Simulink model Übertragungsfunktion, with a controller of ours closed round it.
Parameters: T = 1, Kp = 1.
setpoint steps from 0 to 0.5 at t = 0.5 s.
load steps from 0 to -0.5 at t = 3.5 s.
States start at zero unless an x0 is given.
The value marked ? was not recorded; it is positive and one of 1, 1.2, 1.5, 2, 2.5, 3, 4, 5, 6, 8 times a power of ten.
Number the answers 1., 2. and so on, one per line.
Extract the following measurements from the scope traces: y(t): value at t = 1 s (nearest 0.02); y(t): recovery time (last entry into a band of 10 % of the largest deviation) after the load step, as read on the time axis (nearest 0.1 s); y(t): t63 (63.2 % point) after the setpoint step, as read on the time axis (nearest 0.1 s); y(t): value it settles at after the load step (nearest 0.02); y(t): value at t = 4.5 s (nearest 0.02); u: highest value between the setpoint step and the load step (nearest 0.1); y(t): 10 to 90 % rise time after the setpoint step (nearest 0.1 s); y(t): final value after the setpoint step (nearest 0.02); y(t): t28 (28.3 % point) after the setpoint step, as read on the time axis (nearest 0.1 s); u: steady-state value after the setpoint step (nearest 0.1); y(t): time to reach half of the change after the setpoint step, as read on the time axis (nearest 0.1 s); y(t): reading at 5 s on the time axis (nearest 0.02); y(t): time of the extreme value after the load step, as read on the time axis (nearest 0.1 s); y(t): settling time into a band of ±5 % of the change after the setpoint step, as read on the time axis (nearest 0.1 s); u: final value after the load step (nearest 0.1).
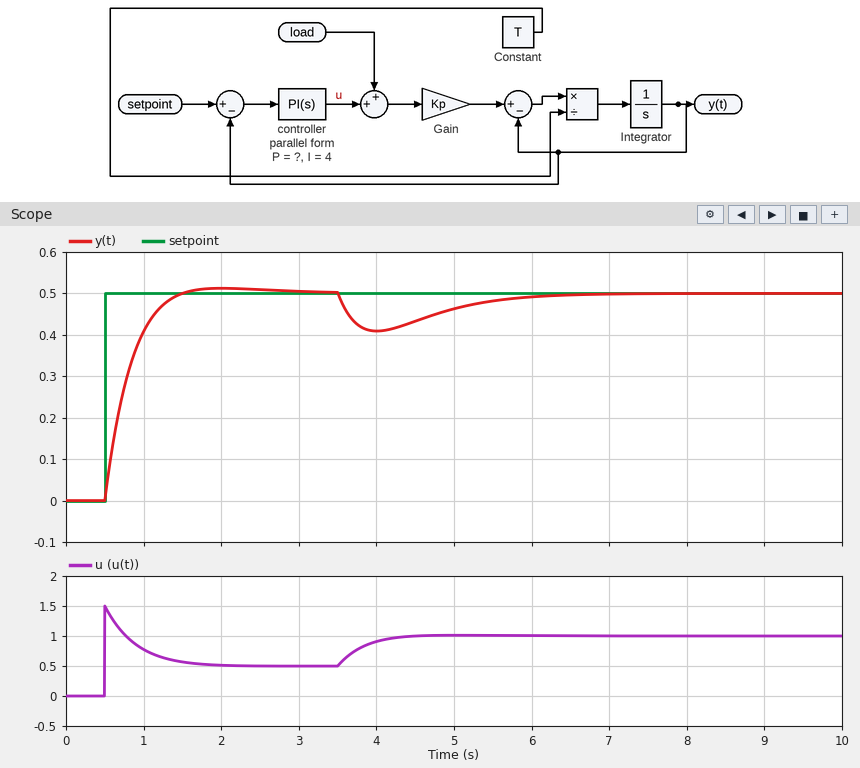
1. 0.40
2. 5.9 s
3. 0.8 s
4. 0.50
5. 0.44
6. 1.5
7. 0.6 s
8. 0.50
9. 0.6 s
10. 0.5
11. 0.7 s
12. 0.46
13. 4.0 s
14. 1.3 s
15. 1.0
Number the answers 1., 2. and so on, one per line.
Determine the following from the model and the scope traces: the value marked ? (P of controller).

1. 3
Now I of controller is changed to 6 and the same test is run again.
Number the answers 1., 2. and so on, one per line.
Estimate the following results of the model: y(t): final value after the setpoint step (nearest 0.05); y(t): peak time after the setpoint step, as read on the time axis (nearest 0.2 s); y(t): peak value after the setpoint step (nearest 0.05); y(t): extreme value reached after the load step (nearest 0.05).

1. 0.50
2. 1.6 s
3. 0.55
4. 0.40
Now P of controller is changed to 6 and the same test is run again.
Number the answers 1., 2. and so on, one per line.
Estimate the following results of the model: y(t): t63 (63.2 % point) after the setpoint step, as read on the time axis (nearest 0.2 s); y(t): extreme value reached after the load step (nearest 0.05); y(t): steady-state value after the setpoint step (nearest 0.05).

1. 0.6 s
2. 0.45
3. 0.50
